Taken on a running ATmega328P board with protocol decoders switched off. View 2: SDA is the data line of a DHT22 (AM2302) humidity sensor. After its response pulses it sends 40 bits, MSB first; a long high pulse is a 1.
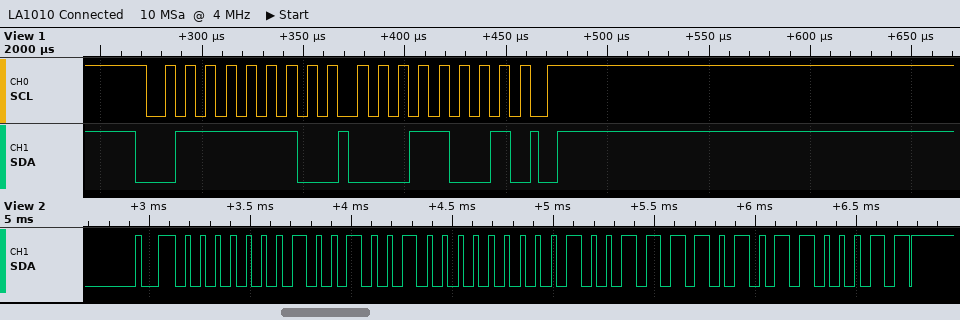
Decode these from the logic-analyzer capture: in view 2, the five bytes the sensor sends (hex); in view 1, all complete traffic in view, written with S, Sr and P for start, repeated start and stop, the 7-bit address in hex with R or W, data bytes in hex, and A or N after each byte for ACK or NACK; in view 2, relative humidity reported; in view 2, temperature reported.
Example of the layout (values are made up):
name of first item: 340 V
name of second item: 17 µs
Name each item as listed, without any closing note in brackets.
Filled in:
in view 2, the five bytes the sensor sends: 01 24 01 3D 63
in view 1, all complete traffic in view, written with S, Sr and P for start, repeated start and stop, the 7-bit address in hex with R or W, data bytes in hex, and A or N after each byte for ACK or NACK: S 3FW A 19 A P
in view 2, relative humidity reported: 29.2 %
in view 2, temperature reported: 31.7 °C
